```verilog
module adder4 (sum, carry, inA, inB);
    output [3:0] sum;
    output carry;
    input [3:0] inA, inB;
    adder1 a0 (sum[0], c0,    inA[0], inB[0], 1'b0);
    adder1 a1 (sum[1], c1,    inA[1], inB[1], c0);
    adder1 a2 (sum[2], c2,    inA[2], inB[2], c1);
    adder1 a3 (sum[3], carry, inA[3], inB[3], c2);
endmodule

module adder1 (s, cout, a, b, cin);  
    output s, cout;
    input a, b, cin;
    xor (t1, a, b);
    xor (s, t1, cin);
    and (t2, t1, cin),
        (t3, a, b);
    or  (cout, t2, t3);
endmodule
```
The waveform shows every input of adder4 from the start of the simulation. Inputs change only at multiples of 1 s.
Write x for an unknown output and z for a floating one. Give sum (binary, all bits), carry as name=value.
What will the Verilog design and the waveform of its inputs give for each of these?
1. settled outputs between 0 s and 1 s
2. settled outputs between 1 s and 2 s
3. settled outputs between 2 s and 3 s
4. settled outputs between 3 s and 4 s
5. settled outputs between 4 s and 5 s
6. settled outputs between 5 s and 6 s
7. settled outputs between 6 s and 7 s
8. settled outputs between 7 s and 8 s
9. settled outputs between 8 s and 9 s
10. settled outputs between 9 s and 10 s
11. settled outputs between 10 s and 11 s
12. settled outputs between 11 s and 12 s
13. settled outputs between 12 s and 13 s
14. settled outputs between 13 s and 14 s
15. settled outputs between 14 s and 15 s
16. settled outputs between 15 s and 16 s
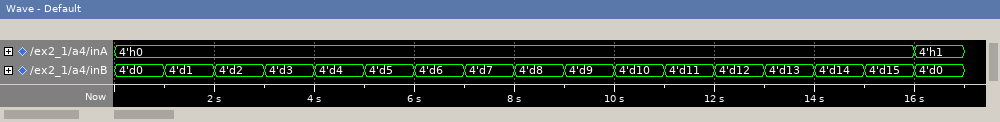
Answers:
sum=0000, carry=0
sum=0001, carry=0
sum=0010, carry=0
sum=0011, carry=0
sum=0100, carry=0
sum=0101, carry=0
sum=0110, carry=0
sum=0111, carry=0
sum=1000, carry=0
sum=1001, carry=0
sum=1010, carry=0
sum=1011, carry=0
sum=1100, carry=0
sum=1101, carry=0
sum=1110, carry=0
sum=1111, carry=0
